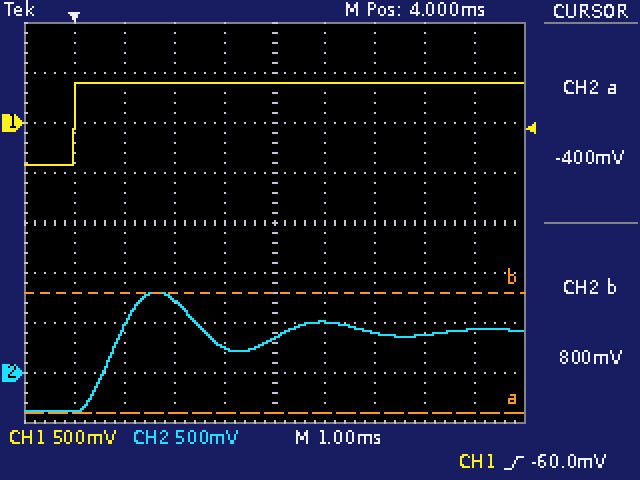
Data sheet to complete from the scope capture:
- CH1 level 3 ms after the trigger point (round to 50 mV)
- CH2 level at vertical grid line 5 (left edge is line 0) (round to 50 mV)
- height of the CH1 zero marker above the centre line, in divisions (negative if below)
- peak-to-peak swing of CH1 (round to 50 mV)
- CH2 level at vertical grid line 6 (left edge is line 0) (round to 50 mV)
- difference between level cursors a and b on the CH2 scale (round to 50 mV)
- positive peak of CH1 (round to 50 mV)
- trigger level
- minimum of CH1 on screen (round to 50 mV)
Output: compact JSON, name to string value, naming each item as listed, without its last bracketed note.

{"CH1 level 3 ms after the trigger point": "400 mV", "CH2 level at vertical grid line 5 (left edge is line 0)": "350 mV", "height of the CH1 zero marker above the centre line, in divisions": "+2.0 div", "peak-to-peak swing of CH1": "800 mV", "CH2 level at vertical grid line 6 (left edge is line 0)": "500 mV", "difference between level cursors a and b on the CH2 scale": "1.20 V", "positive peak of CH1": "400 mV", "trigger level": "-60.0 mV", "minimum of CH1 on screen": "-400 mV"}
